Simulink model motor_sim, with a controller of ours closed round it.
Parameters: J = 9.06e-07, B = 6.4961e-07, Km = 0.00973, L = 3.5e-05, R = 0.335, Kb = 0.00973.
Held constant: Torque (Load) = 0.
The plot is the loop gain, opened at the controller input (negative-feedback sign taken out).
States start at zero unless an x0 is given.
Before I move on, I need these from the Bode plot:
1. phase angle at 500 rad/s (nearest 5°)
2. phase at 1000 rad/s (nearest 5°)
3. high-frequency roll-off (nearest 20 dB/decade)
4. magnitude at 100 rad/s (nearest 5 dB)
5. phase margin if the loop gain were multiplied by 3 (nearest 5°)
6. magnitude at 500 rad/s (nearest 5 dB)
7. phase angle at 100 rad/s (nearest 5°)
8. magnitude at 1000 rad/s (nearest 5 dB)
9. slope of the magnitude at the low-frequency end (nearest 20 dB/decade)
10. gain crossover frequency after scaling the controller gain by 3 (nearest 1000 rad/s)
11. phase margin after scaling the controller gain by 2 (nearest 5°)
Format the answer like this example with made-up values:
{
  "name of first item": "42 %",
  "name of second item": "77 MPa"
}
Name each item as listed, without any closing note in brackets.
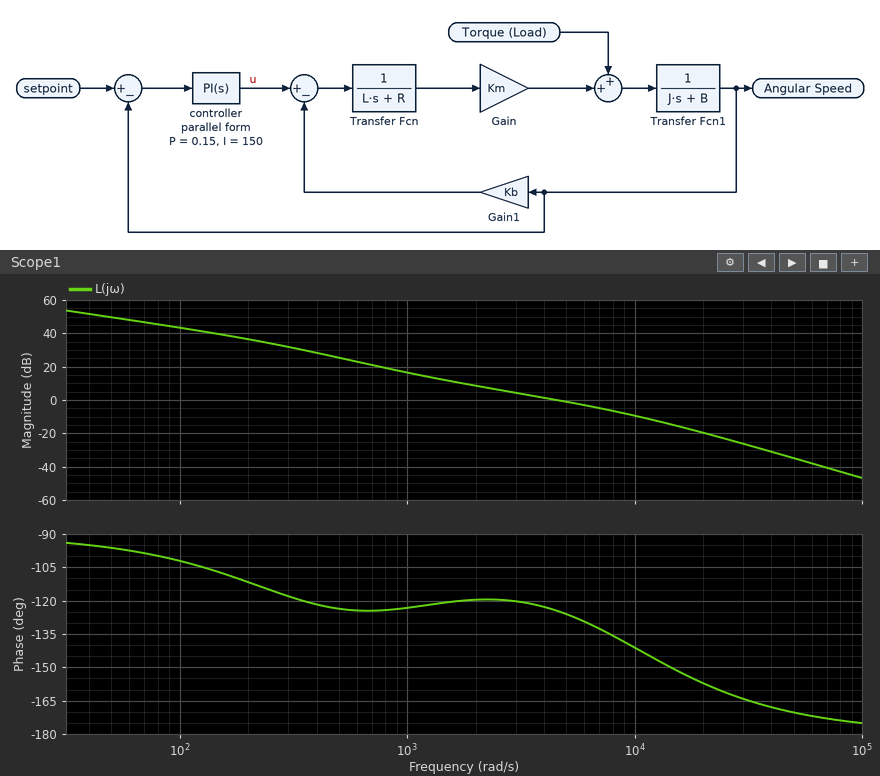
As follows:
{
  "phase angle at 500 rad/s": "-125°",
  "phase at 1000 rad/s": "-125°",
  "high-frequency roll-off": "-40 dB/decade",
  "magnitude at 100 rad/s": "45 dB",
  "phase margin if the loop gain were multiplied by 3": "40°",
  "magnitude at 500 rad/s": "25 dB",
  "phase angle at 100 rad/s": "-100°",
  "magnitude at 1000 rad/s": "15 dB",
  "slope of the magnitude at the low-frequency end": "-20 dB/decade",
  "gain crossover frequency after scaling the controller gain by 3": "10000 rad/s",
  "phase margin after scaling the controller gain by 2": "45°"
}
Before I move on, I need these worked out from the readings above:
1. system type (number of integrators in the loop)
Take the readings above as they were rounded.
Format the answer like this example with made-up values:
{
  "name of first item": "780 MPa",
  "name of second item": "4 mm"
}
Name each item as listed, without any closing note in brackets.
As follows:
{
  "system type": "1"
}
